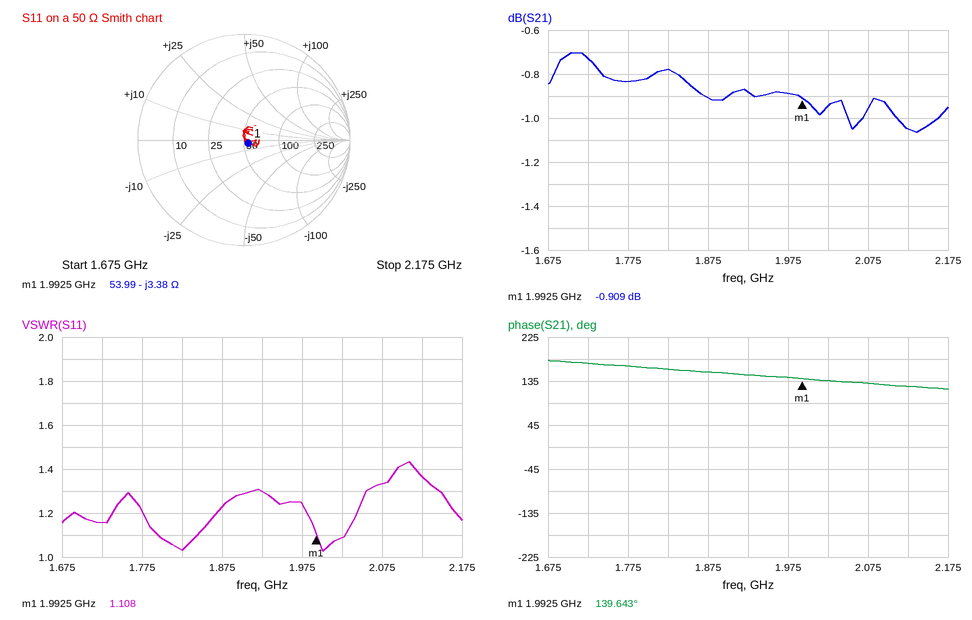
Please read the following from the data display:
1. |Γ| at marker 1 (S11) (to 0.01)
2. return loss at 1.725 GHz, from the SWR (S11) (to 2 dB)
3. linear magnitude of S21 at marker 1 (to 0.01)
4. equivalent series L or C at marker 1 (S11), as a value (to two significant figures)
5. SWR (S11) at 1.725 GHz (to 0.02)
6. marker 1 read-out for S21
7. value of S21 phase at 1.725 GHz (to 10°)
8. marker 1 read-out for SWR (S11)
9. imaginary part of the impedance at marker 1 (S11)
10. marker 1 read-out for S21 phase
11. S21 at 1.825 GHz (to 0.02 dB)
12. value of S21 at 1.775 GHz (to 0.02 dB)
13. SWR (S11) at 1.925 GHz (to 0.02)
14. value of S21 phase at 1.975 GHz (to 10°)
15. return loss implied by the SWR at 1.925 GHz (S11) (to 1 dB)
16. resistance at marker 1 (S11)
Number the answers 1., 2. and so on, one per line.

1. 0.05
2. 22 dB
3. 0.90
4. 24 pF
5. 1.16
6. -0.909 dB
7. 170°
8. 1.108
9. -3.38 Ω
10. 139.643°
11. -0.78 dB
12. -0.84 dB
13. 1.30
14. 140°
15. 18 dB
16. 53.99 Ω
